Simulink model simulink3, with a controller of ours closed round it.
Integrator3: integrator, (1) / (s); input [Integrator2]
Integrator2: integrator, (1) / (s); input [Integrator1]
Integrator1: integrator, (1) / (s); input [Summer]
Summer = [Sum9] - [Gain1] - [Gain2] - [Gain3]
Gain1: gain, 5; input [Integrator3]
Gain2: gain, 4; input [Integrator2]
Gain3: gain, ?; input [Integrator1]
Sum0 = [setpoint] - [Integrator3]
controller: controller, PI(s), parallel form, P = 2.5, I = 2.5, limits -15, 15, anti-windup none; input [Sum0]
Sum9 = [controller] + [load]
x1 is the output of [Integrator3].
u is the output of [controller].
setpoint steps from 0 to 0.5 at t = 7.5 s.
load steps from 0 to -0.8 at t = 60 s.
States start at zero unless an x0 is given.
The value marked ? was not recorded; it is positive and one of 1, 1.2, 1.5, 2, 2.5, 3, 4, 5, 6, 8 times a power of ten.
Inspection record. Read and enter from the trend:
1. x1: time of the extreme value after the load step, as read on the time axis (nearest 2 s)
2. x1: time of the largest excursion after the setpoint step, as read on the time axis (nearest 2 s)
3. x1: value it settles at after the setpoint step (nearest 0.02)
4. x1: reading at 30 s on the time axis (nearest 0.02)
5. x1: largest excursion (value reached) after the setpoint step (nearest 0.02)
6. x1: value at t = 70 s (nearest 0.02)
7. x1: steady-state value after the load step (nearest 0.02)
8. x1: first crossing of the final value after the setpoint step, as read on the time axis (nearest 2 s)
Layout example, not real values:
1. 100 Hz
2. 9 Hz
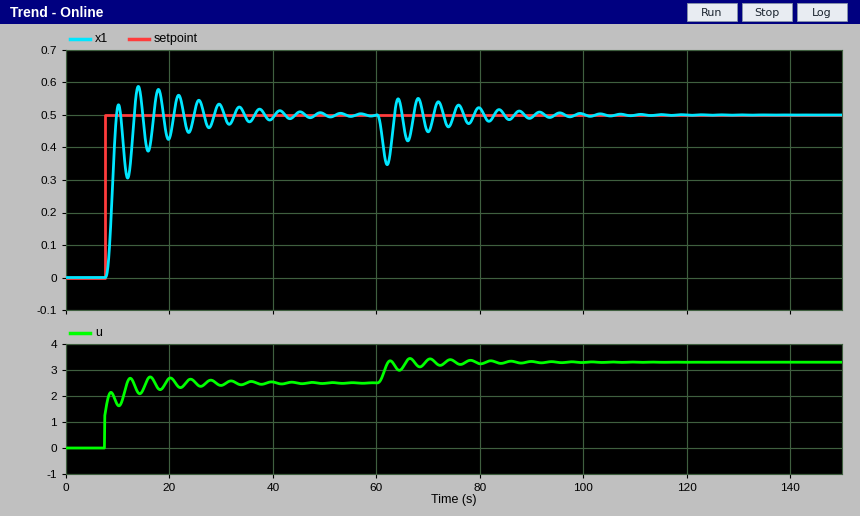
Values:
1. 62 s
2. 14 s
3. 0.50
4. 0.52
5. 0.58
6. 0.44
7. 0.50
8. 10 s
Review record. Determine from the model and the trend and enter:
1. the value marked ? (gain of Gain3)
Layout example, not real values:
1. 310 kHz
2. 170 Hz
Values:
1. 3
